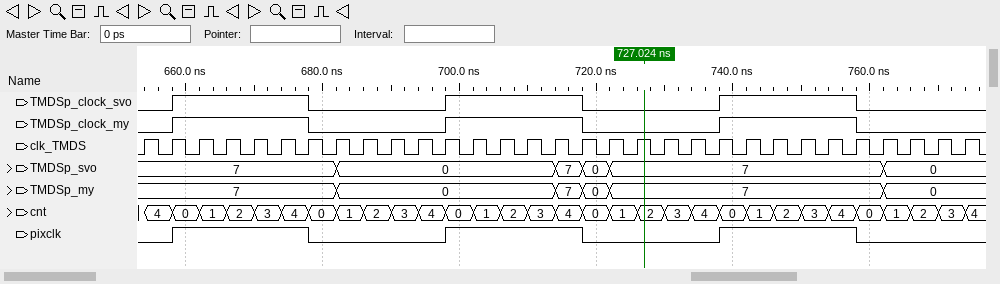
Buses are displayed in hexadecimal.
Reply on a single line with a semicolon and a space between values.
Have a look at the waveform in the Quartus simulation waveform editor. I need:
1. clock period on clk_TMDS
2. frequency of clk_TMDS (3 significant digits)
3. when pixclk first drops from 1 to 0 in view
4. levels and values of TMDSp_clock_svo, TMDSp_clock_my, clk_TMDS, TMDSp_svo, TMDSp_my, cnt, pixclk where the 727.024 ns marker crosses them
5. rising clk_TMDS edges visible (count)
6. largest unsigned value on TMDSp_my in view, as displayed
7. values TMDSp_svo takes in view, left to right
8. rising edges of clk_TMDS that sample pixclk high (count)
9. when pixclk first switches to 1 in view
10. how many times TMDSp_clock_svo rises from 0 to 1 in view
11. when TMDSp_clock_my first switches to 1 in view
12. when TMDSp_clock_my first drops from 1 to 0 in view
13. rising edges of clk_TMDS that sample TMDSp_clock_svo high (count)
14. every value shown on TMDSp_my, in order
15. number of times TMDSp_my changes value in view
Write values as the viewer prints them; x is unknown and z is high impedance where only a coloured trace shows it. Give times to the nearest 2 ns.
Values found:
4 ns; 250 MHz; 678 ns; TMDSp_clock_svo=0, TMDSp_clock_my=0, clk_TMDS=1, TMDSp_svo=7, TMDSp_my=7, cnt=2, pixclk=0; 31; 7; 7, 0, 7, 0, 7, 0; 15; 658 ns; 3; 658 ns; 678 ns; 15; 7, 0, 7, 0, 7, 0; 5
